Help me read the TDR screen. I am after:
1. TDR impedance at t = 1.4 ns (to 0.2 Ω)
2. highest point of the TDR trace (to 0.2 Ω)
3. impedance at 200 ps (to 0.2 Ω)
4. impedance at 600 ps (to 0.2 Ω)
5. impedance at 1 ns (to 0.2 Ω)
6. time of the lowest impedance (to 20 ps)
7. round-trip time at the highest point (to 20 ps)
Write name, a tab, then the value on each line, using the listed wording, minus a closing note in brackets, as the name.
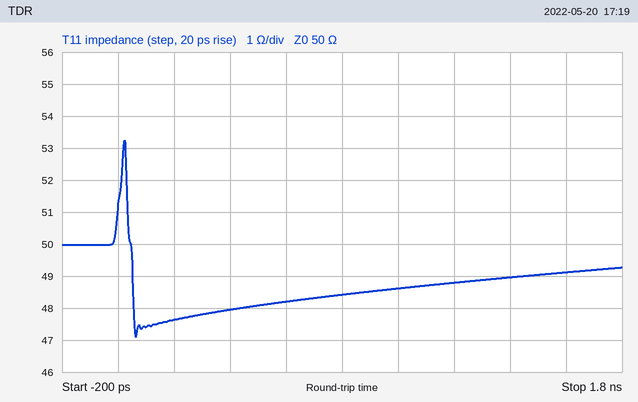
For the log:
TDR impedance at t = 1.4 ns	49.0 Ω
highest point of the TDR trace	53.2 Ω
impedance at 200 ps	47.6 Ω
impedance at 600 ps	48.2 Ω
impedance at 1 ns	48.6 Ω
time of the lowest impedance	60 ps
round-trip time at the highest point	20 ps
